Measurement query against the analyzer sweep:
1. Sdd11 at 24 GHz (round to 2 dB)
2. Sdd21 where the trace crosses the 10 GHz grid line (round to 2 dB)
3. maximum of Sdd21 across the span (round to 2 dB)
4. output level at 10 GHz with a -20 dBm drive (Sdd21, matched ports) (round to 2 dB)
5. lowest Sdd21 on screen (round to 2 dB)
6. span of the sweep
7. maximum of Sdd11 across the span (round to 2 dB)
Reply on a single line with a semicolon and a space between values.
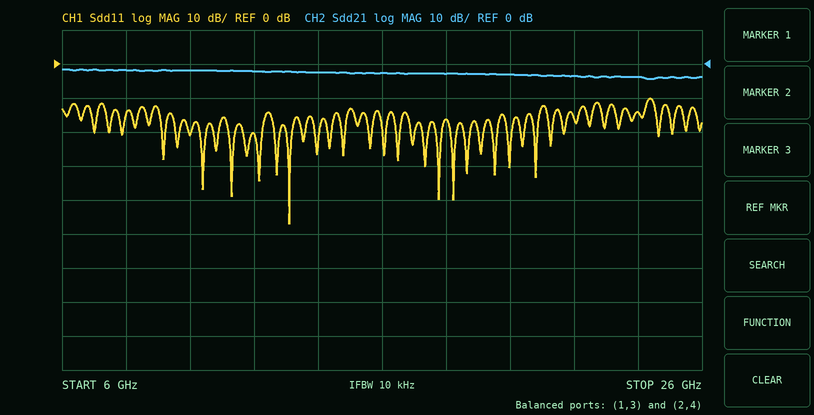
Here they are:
-14 dB; -2 dB; -2 dB; -22 dBm; -4 dB; 20 GHz; -10 dB
